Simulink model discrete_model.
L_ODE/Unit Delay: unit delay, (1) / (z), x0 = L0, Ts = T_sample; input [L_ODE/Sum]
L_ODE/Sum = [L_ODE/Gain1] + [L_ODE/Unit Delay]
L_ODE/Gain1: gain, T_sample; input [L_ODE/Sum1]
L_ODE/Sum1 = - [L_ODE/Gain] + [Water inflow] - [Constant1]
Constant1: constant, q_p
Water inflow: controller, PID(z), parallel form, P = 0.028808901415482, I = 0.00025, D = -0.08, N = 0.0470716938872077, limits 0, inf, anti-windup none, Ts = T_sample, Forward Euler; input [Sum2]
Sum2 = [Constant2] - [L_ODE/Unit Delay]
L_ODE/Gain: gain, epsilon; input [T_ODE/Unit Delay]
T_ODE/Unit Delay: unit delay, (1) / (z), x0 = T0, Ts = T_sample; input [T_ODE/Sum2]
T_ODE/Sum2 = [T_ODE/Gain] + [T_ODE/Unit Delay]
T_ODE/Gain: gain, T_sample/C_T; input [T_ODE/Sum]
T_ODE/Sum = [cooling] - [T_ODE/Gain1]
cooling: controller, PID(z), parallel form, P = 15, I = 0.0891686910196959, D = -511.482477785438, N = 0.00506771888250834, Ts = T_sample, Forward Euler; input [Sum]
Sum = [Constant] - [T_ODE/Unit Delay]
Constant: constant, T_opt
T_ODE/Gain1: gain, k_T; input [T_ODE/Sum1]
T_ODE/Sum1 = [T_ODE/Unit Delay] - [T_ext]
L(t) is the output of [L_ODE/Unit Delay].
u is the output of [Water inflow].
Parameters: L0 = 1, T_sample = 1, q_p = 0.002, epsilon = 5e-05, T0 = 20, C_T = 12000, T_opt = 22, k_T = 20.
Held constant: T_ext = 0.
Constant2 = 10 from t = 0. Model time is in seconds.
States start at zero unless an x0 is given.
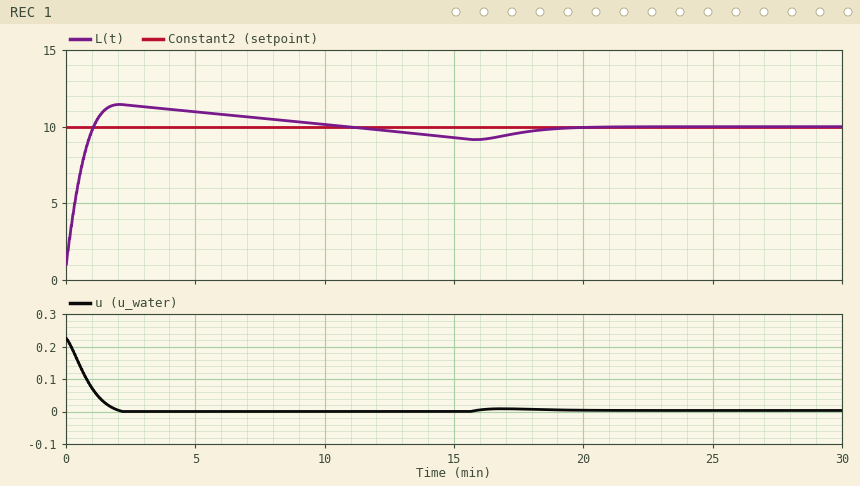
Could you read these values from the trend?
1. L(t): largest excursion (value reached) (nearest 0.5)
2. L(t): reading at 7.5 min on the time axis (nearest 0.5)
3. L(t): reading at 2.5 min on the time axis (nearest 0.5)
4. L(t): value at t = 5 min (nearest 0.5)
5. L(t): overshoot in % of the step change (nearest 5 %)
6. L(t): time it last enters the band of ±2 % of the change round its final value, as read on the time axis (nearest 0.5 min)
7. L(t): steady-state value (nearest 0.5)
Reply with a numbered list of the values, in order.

1. 11.5
2. 10.5
3. 11.5
4. 11.0
5. 15 %
6. 18.5 min
7. 10.0
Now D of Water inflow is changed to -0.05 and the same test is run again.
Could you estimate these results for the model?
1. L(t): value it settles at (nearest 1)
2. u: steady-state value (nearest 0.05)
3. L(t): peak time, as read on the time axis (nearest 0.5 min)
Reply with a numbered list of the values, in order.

1. 10
2. 0.00
3. 2.0 min
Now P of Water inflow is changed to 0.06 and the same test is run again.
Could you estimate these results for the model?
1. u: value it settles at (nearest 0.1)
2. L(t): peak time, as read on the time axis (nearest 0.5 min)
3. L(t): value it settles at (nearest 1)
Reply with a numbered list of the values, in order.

1. 0.0
2. 1.5 min
3. 10
